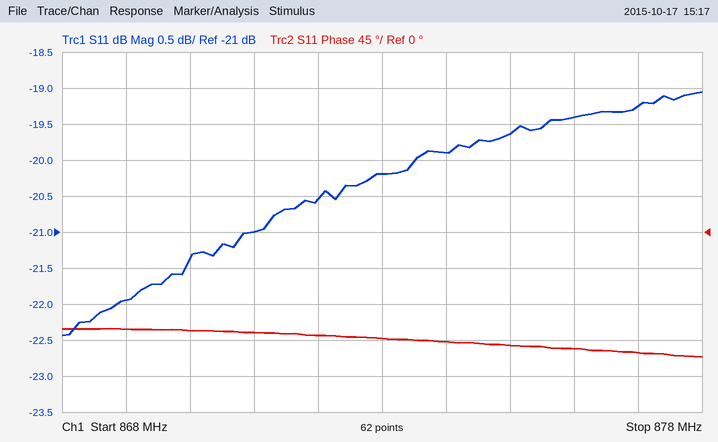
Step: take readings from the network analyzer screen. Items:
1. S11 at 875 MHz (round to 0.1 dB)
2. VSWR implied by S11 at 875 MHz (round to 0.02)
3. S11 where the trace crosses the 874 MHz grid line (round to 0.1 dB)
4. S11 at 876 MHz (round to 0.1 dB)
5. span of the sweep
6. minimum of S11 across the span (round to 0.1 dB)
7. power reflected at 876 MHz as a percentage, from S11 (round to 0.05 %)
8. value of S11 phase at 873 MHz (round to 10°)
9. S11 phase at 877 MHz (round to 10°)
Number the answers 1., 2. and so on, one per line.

1. -19.6 dB
2. 1.24
3. -19.9 dB
4. -19.4 dB
5. 10 MHz
6. -22.4 dB
7. 1.15 %
8. -130°
9. -150°
